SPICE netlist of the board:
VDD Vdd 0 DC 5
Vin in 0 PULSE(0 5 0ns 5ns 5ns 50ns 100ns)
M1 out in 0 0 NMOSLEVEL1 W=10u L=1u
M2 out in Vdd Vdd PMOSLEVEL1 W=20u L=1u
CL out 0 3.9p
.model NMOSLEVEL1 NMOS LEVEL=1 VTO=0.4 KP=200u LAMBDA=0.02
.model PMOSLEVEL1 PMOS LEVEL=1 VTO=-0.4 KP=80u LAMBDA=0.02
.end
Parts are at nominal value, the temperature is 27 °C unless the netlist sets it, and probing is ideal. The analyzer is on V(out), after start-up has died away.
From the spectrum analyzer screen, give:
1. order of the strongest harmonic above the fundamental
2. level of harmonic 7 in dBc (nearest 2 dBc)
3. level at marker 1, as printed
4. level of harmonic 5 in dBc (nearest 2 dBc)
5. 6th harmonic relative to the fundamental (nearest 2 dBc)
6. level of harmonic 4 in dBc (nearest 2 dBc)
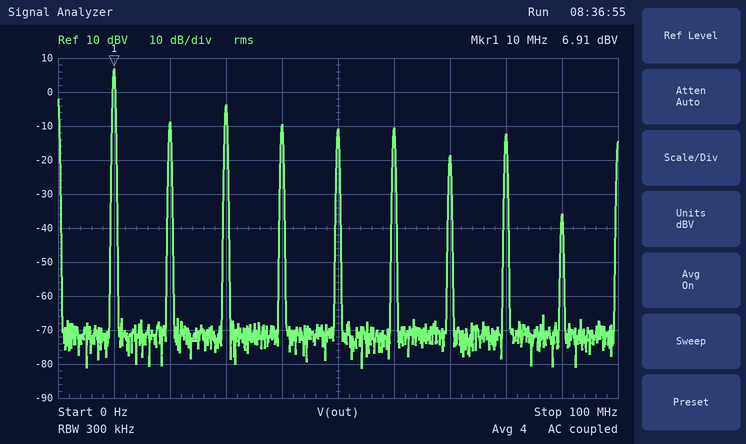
3
-26 dBc
6.91 dBV
-18 dBc
-18 dBc
-16 dBc
